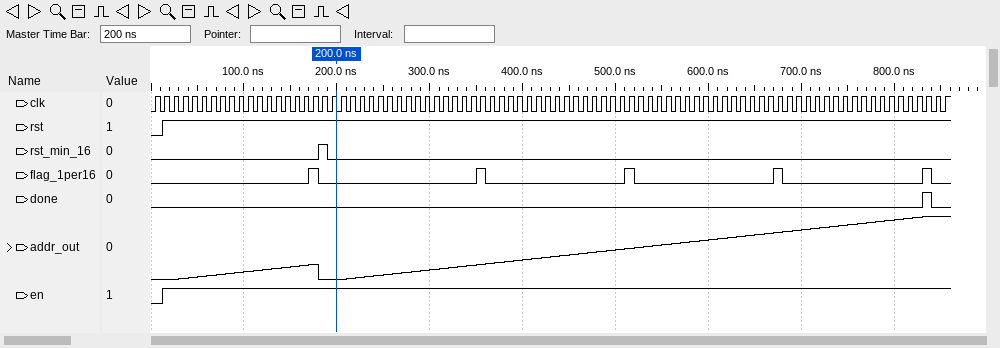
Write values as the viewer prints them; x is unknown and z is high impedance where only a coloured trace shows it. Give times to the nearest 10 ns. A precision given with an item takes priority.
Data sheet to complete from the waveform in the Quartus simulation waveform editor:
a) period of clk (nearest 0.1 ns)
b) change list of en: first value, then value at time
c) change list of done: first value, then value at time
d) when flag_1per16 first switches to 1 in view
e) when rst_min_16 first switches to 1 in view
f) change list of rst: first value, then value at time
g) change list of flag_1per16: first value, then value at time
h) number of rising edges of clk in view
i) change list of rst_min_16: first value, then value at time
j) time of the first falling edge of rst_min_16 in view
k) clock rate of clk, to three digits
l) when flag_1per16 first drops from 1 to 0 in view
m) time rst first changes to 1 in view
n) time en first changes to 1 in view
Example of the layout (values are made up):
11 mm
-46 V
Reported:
10 ns
0, 1 at 10 ns
0, 1 at 830 ns, 0 at 840 ns
170 ns
180 ns
0, 1 at 10 ns
0, 1 at 170 ns, 0 at 180 ns, 1 at 350 ns, 0 at 360 ns, 1 at 510 ns, 0 at 520 ns, 1 at 670 ns, 0 at 680 ns, 1 at 830 ns, 0 at 840 ns
86
0, 1 at 180 ns, 0 at 190 ns
190 ns
100 MHz
180 ns
10 ns
10 ns
